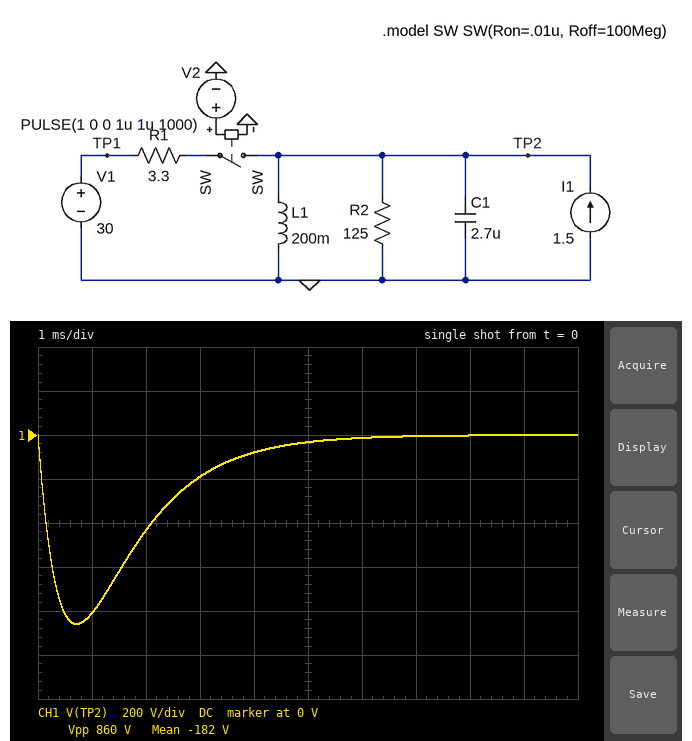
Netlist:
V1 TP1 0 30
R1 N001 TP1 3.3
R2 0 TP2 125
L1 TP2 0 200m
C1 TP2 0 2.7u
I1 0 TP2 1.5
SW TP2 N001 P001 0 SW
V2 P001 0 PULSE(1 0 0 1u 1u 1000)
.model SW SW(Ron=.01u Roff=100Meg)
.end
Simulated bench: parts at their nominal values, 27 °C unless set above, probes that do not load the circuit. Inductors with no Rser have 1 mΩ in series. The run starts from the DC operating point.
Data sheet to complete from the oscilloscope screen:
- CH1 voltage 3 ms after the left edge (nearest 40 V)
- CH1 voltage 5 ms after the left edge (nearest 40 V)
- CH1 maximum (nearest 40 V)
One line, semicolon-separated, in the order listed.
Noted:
-200 V; -40 V; 0 V
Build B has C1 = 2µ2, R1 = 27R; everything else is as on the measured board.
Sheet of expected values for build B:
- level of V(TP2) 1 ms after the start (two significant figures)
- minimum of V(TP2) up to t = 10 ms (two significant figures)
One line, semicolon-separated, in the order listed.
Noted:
-97 V; -110 V
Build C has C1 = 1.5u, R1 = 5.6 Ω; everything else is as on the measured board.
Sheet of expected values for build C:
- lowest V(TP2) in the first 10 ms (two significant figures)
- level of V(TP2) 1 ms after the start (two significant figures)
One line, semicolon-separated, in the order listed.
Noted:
-550 V; -440 V
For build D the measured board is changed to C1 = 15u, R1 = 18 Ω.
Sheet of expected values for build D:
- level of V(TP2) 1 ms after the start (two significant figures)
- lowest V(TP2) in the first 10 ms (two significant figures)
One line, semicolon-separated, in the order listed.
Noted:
-81 V; -110 V
